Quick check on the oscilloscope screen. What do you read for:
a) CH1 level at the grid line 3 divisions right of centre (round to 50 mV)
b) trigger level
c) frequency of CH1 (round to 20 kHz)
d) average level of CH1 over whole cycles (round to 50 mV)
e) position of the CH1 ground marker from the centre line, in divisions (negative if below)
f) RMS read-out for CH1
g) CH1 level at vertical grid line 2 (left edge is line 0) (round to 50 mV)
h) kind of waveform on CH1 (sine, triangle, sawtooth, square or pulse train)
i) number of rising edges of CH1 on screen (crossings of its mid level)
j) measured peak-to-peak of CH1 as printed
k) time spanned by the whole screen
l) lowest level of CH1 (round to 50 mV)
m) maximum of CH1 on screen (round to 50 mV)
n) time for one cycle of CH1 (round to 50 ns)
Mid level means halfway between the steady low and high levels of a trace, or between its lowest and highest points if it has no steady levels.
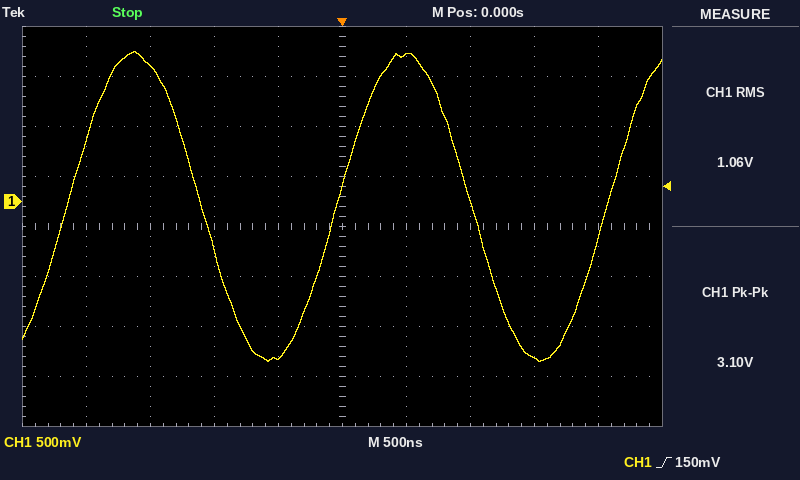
-1.55 V
150 mV
480 kHz
-50 mV
+0.5 div
1.06 V
1.35 V
sine
3
3.10 V
5 µs
-1.60 V
1.50 V
2.10 µs
